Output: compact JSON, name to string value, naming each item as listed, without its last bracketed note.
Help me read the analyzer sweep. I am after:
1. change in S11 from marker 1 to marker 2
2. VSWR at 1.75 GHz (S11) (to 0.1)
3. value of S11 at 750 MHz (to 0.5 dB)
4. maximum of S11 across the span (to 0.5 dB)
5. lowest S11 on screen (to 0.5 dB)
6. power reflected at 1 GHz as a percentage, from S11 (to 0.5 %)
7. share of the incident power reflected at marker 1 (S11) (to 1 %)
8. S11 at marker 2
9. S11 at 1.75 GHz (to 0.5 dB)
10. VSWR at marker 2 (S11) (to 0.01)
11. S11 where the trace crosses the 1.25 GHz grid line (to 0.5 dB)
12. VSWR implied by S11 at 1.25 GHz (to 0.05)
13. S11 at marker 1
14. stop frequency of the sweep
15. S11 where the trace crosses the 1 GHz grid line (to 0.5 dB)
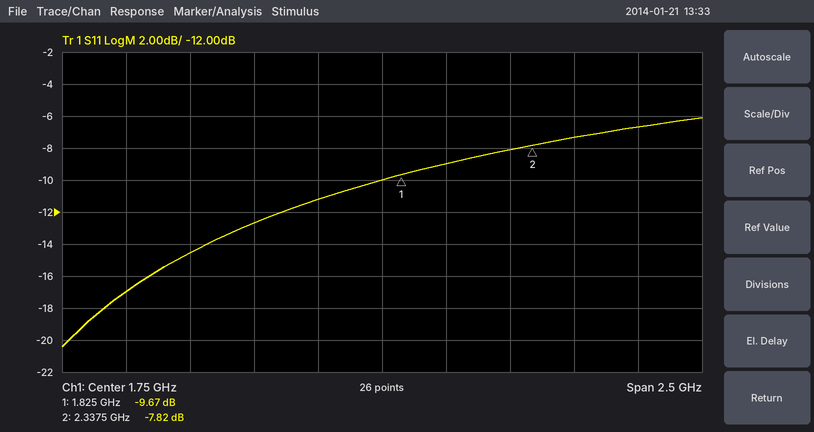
{"change in S11 from marker 1 to marker 2": "1.85 dB", "VSWR at 1.75 GHz (S11)": "1.9", "value of S11 at 750 MHz": "-17.0 dB", "maximum of S11 across the span": "-6.0 dB", "lowest S11 on screen": "-20.5 dB", "power reflected at 1 GHz as a percentage, from S11": "3.5 %", "share of the incident power reflected at marker 1 (S11)": "11 %", "S11 at marker 2": "-7.82 dB", "S11 at 1.75 GHz": "-10.0 dB", "VSWR at marker 2 (S11)": "2.37", "S11 where the trace crosses the 1.25 GHz grid line": "-12.5 dB", "VSWR implied by S11 at 1.25 GHz": "1.60", "S11 at marker 1": "-9.67 dB", "stop frequency of the sweep": "3 GHz", "S11 where the trace crosses the 1 GHz grid line": "-14.5 dB"}
